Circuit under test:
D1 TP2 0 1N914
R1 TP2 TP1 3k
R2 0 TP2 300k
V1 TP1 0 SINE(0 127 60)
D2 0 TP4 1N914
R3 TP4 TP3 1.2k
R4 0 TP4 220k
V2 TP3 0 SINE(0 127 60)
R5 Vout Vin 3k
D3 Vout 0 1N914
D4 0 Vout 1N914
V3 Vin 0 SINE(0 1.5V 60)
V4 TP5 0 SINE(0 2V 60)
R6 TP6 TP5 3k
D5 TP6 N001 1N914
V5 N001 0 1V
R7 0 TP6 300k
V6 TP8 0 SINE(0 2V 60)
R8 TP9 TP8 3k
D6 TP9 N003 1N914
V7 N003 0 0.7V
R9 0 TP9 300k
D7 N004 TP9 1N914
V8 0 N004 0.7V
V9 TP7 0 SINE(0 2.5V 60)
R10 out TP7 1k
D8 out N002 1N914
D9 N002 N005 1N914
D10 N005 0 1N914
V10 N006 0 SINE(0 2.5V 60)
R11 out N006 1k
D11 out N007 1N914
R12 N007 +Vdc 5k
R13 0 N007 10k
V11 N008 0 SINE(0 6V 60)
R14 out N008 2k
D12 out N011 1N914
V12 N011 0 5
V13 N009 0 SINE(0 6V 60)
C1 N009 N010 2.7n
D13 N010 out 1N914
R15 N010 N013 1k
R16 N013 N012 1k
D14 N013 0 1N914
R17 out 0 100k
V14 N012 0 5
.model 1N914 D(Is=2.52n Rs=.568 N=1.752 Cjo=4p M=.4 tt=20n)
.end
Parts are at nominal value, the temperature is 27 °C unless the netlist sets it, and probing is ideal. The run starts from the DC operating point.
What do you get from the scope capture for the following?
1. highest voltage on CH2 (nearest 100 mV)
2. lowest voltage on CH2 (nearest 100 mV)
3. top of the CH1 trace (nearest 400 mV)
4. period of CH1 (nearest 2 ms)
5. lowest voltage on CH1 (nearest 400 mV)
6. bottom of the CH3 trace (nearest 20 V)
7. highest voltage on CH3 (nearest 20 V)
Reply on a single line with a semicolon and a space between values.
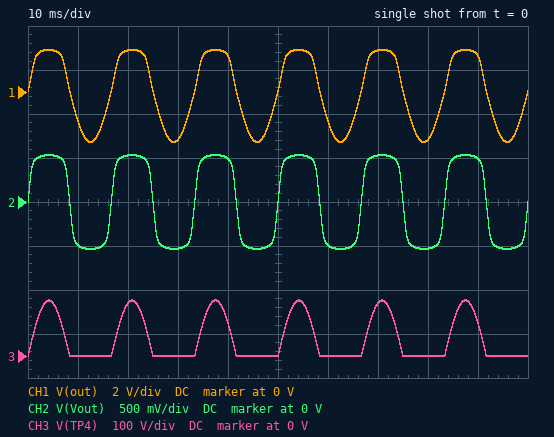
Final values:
500 mV; -500 mV; 2.0 V; 16 ms; -2.4 V; 0 V; 120 V
